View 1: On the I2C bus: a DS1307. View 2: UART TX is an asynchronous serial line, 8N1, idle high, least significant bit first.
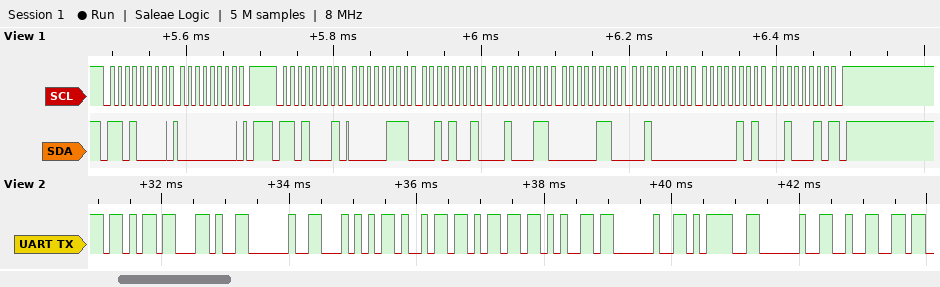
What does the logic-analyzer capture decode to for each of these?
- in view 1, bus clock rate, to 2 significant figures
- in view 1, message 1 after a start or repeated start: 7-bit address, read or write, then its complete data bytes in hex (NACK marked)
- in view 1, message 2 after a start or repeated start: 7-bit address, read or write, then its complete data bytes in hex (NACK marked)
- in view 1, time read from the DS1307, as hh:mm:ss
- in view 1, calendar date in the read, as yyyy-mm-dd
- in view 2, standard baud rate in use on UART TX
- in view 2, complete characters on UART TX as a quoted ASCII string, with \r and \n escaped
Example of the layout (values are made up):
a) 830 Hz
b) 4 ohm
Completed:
a) 100 kHz
b) 0x68 write: 00
c) 0x68 read: 07 29 23 06 20 05 22 NACK
d) 23:29:07
e) 2022-05-20
f) 9600 baud
g) "k, Time = 2"
